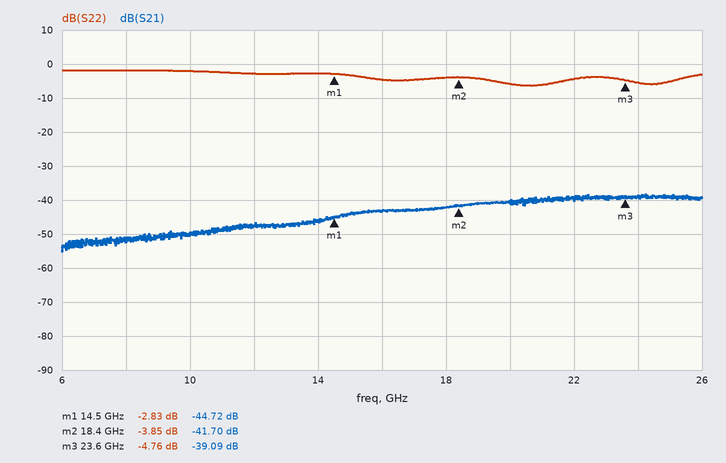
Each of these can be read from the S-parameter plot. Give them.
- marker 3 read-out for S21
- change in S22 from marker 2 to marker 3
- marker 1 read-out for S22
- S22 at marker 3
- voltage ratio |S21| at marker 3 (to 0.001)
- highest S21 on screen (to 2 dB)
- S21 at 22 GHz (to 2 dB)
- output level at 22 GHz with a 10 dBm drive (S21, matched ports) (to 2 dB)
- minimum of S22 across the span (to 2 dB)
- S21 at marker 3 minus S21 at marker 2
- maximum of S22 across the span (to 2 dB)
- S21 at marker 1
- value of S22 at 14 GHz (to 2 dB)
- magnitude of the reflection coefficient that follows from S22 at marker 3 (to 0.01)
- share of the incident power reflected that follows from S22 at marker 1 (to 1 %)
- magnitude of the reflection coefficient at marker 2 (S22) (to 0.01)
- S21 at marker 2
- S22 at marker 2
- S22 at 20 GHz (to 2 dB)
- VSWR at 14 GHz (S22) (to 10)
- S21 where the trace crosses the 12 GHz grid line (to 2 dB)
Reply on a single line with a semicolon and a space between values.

-39.09 dB; -0.91 dB; -2.83 dB; -4.76 dB; 0.011; -38 dB; -40 dB; -30 dBm; -6 dB; 2.61 dB; -2 dB; -44.72 dB; -2 dB; 0.58; 52 %; 0.64; -41.70 dB; -3.85 dB; -6 dB; 10; -48 dB
